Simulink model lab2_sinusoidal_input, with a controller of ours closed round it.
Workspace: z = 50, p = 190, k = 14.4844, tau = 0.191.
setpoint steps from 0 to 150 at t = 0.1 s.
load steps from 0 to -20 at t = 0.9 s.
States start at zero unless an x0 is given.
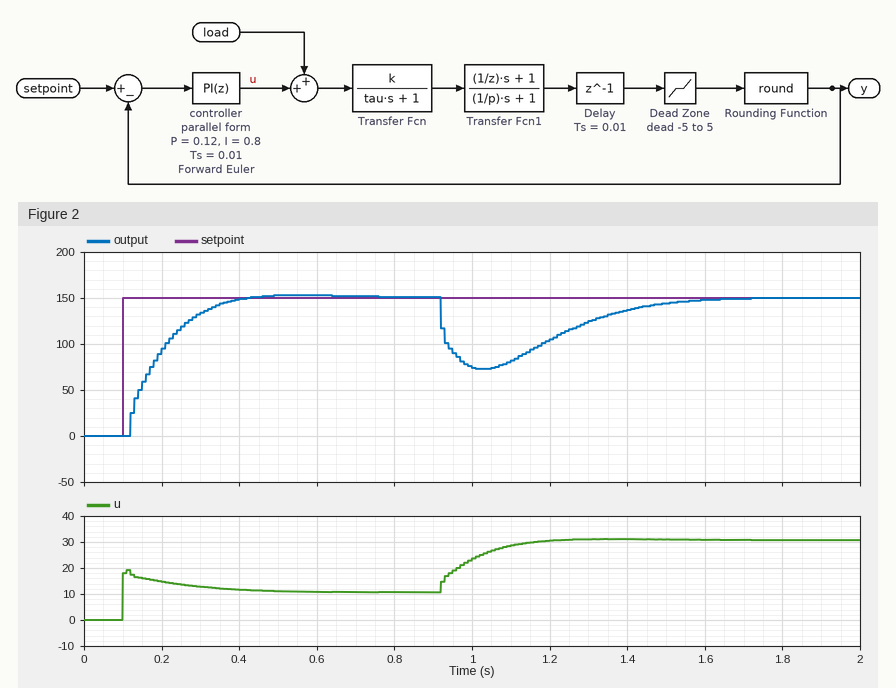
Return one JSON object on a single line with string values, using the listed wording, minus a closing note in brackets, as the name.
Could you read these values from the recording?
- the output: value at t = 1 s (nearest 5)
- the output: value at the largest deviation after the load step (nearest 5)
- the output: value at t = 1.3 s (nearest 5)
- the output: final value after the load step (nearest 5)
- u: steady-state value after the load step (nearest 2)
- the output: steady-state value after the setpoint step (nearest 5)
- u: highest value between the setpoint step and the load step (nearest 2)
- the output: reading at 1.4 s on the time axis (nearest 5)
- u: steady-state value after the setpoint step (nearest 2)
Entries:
{"the output: value at t = 1 s": "75", "the output: value at the largest deviation after the load step": "75", "the output: value at t = 1.3 s": "125", "the output: final value after the load step": "150", "u: steady-state value after the load step": "30", "the output: steady-state value after the setpoint step": "150", "u: highest value between the setpoint step and the load step": "20", "the output: reading at 1.4 s on the time axis": "135", "u: steady-state value after the setpoint step": "10"}
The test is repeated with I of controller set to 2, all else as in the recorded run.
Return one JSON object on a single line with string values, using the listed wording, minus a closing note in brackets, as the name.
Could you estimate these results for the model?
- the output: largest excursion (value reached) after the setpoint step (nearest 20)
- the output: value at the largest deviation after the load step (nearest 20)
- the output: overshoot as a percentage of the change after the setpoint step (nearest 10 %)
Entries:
{"the output: largest excursion (value reached) after the setpoint step": "180", "the output: value at the largest deviation after the load step": "80", "the output: overshoot as a percentage of the change after the setpoint step": "20 %"}
